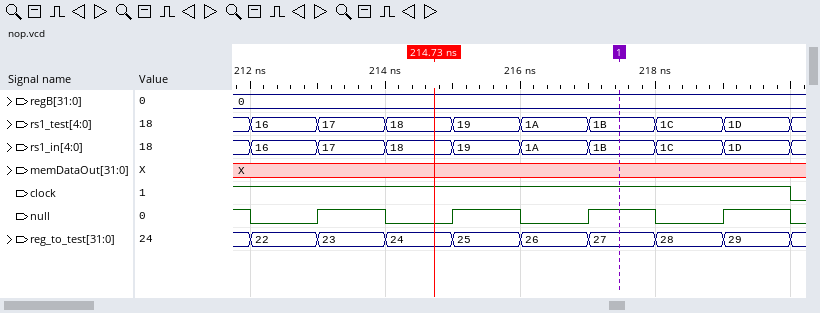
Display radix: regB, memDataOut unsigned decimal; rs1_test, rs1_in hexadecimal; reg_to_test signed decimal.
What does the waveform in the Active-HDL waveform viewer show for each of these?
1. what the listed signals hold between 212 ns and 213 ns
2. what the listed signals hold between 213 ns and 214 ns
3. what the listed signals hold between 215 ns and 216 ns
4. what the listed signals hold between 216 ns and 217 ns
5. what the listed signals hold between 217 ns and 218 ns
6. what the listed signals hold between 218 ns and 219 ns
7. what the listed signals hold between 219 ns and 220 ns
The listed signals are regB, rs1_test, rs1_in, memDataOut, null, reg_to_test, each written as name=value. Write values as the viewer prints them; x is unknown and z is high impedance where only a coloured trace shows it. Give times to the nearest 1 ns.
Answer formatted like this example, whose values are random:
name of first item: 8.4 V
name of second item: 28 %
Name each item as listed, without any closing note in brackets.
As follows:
what the listed signals hold between 212 ns and 213 ns: regB=0, rs1_test=16, rs1_in=16, memDataOut=X, null=0, reg_to_test=22
what the listed signals hold between 213 ns and 214 ns: regB=0, rs1_test=17, rs1_in=17, memDataOut=X, null=1, reg_to_test=23
what the listed signals hold between 215 ns and 216 ns: regB=0, rs1_test=19, rs1_in=19, memDataOut=X, null=1, reg_to_test=25
what the listed signals hold between 216 ns and 217 ns: regB=0, rs1_test=1A, rs1_in=1A, memDataOut=X, null=0, reg_to_test=26
what the listed signals hold between 217 ns and 218 ns: regB=0, rs1_test=1B, rs1_in=1B, memDataOut=X, null=1, reg_to_test=27
what the listed signals hold between 218 ns and 219 ns: regB=0, rs1_test=1C, rs1_in=1C, memDataOut=X, null=0, reg_to_test=28
what the listed signals hold between 219 ns and 220 ns: regB=0, rs1_test=1D, rs1_in=1D, memDataOut=X, null=1, reg_to_test=29
